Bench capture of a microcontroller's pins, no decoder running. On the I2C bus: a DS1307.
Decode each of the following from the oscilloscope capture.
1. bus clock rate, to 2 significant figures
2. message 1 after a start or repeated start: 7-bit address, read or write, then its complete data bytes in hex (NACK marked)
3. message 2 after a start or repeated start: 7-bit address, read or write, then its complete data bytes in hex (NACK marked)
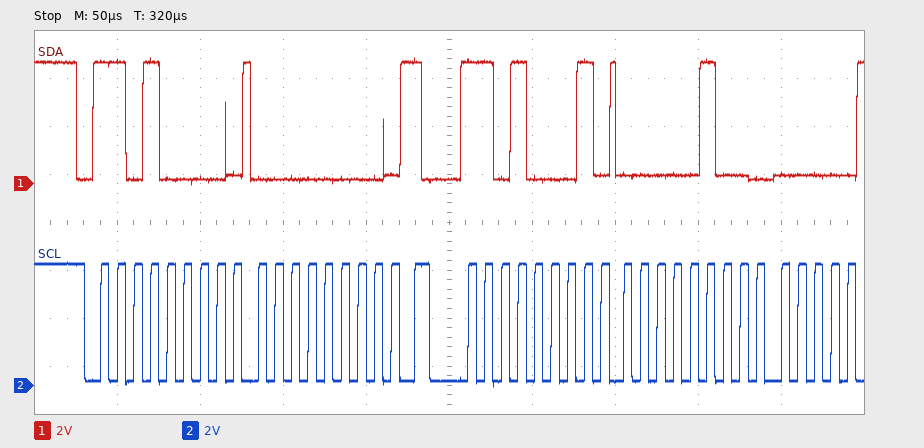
100 kHz
0x68 write: 00
0x68 read: 04
